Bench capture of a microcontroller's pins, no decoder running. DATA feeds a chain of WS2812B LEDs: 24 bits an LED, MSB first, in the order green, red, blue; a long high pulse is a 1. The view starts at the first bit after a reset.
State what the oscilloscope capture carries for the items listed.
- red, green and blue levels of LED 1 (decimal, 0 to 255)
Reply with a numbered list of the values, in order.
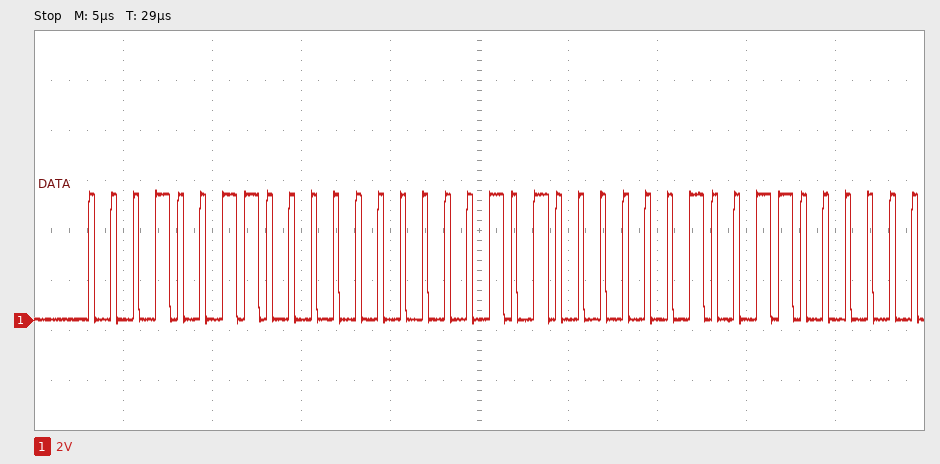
1. 0, 19, 40
